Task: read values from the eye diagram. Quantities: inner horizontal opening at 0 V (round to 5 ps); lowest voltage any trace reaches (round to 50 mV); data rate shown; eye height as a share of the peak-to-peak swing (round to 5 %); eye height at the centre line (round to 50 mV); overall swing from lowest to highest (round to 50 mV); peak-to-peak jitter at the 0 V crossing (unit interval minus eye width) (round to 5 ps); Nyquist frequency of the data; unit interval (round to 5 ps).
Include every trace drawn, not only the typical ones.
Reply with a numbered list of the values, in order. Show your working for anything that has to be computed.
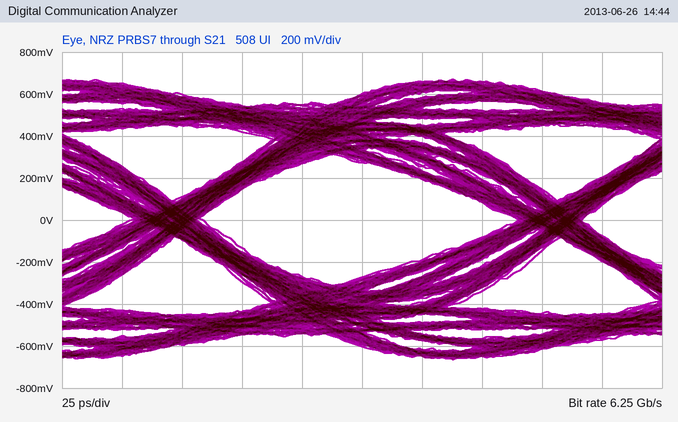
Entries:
1. 130 ps
2. -650 mV
3. 6.25 Gb/s
4. 550 mV / 1.35 V ≈ 40.7 %, so 40 % to the nearest 5 %
5. 550 mV
6. 1.35 V
7. 30 ps
8. 3.125 GHz
9. 160 ps
